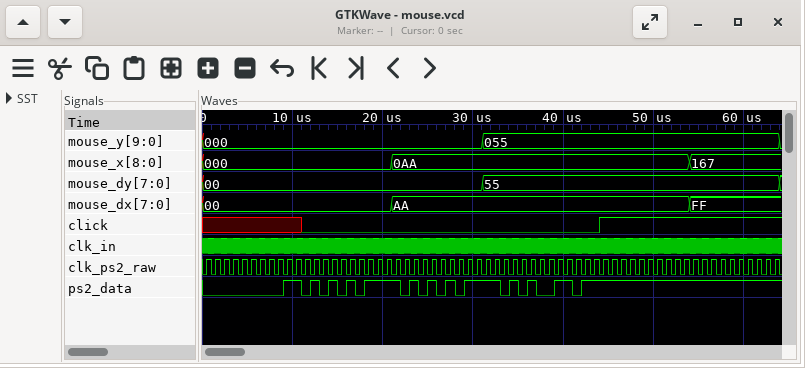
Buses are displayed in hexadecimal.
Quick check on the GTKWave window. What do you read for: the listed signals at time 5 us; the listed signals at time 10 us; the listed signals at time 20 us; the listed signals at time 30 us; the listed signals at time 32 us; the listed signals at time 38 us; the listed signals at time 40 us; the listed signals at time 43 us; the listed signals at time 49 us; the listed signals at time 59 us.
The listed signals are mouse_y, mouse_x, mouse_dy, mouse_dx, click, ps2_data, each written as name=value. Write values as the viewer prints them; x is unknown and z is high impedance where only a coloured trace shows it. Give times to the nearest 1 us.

mouse_y=000, mouse_x=000, mouse_dy=00, mouse_dx=00, click=x, ps2_data=0
mouse_y=000, mouse_x=000, mouse_dy=00, mouse_dx=00, click=x, ps2_data=1
mouse_y=000, mouse_x=000, mouse_dy=00, mouse_dx=00, click=0, ps2_data=1
mouse_y=000, mouse_x=0AA, mouse_dy=00, mouse_dx=AA, click=0, ps2_data=1
mouse_y=055, mouse_x=0AA, mouse_dy=55, mouse_dx=AA, click=0, ps2_data=1
mouse_y=055, mouse_x=0AA, mouse_dy=55, mouse_dx=AA, click=0, ps2_data=0
mouse_y=055, mouse_x=0AA, mouse_dy=55, mouse_dx=AA, click=0, ps2_data=1
mouse_y=055, mouse_x=0AA, mouse_dy=55, mouse_dx=AA, click=0, ps2_data=1
mouse_y=055, mouse_x=0AA, mouse_dy=55, mouse_dx=AA, click=1, ps2_data=1
mouse_y=055, mouse_x=167, mouse_dy=55, mouse_dx=FF, click=1, ps2_data=1
